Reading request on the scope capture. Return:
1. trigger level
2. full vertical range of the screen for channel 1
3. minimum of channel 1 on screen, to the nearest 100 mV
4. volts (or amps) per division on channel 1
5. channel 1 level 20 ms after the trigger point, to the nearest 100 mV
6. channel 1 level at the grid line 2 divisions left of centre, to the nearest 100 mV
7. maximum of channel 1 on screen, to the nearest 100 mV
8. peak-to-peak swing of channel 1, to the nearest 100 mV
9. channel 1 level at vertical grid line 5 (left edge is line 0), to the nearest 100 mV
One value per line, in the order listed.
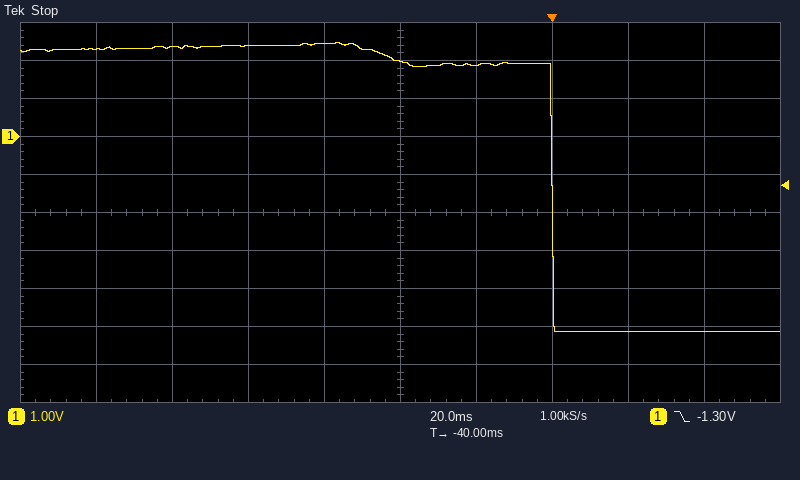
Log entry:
-1.30 V
10 V
-5.1 V
1 V
-5.1 V
2.4 V
2.5 V
7.6 V
2.0 V
